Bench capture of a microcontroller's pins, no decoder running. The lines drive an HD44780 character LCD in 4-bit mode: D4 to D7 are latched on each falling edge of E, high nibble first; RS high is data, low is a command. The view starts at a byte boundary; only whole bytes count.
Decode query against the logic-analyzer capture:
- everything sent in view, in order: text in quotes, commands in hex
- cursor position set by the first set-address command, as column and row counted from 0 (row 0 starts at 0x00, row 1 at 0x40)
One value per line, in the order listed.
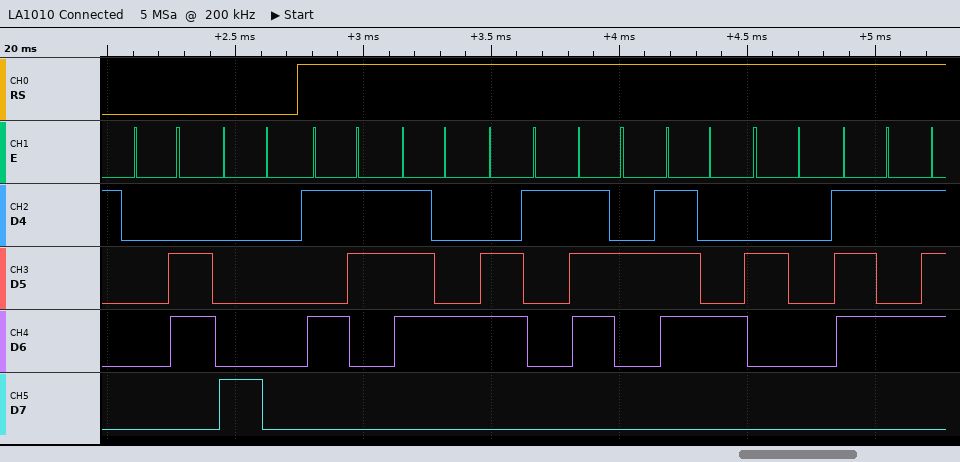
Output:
0x06 0x80 "Start u"
column 0, row 0
